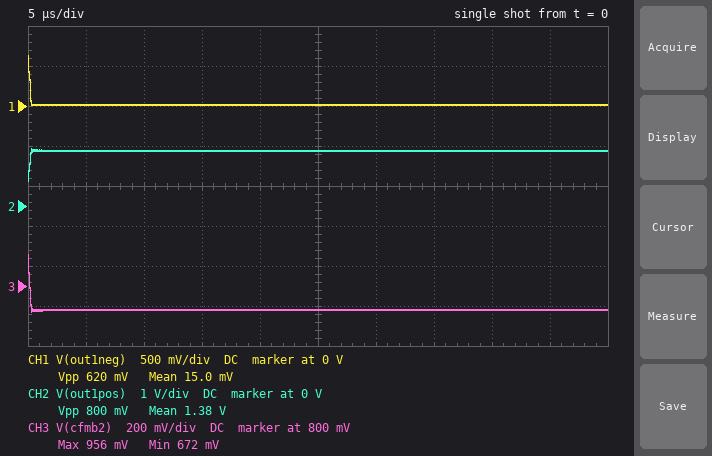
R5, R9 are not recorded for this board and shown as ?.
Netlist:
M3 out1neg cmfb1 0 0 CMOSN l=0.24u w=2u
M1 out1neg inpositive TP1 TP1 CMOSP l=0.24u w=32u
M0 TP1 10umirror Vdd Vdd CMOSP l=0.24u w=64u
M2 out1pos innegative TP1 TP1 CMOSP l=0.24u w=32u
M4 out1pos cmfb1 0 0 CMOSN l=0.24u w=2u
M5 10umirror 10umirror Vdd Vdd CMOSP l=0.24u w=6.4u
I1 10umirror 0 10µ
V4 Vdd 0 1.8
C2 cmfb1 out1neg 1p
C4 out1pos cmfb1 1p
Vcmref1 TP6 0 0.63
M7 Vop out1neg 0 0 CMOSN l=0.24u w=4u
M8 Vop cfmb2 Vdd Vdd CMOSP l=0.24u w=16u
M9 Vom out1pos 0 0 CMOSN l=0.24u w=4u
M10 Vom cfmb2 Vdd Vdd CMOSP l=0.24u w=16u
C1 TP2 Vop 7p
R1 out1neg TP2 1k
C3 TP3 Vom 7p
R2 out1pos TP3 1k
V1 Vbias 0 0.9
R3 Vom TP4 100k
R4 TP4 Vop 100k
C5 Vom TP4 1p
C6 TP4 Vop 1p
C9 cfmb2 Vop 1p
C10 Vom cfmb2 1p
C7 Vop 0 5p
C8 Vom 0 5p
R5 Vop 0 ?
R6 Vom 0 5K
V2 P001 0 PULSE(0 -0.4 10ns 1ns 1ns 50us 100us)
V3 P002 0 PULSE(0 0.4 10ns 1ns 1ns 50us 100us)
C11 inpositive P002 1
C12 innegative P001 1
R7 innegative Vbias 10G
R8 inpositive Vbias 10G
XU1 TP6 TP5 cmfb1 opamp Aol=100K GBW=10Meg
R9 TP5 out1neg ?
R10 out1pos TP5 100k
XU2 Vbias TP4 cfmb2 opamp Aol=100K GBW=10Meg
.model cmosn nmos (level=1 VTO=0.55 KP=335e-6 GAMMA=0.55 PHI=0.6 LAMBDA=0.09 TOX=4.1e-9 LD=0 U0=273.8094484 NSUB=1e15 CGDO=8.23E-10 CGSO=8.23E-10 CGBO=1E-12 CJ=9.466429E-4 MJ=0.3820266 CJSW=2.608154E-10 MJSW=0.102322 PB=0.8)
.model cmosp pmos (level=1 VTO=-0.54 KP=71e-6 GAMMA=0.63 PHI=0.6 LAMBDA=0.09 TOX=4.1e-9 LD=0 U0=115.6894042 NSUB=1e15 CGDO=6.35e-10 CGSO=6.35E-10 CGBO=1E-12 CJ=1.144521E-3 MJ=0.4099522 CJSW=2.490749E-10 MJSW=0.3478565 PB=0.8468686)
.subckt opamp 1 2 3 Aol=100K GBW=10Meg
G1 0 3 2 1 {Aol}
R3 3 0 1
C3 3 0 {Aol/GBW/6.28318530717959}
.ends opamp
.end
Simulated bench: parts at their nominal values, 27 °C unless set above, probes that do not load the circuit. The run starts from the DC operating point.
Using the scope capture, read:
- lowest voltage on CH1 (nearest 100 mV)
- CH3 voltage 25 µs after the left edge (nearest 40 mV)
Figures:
0 V
680 mV
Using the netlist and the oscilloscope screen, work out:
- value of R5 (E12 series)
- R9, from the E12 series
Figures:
3.3 kΩ
82 kΩ
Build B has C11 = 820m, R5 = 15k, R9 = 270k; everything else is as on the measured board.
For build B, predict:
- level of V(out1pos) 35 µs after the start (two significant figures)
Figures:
860 mV
